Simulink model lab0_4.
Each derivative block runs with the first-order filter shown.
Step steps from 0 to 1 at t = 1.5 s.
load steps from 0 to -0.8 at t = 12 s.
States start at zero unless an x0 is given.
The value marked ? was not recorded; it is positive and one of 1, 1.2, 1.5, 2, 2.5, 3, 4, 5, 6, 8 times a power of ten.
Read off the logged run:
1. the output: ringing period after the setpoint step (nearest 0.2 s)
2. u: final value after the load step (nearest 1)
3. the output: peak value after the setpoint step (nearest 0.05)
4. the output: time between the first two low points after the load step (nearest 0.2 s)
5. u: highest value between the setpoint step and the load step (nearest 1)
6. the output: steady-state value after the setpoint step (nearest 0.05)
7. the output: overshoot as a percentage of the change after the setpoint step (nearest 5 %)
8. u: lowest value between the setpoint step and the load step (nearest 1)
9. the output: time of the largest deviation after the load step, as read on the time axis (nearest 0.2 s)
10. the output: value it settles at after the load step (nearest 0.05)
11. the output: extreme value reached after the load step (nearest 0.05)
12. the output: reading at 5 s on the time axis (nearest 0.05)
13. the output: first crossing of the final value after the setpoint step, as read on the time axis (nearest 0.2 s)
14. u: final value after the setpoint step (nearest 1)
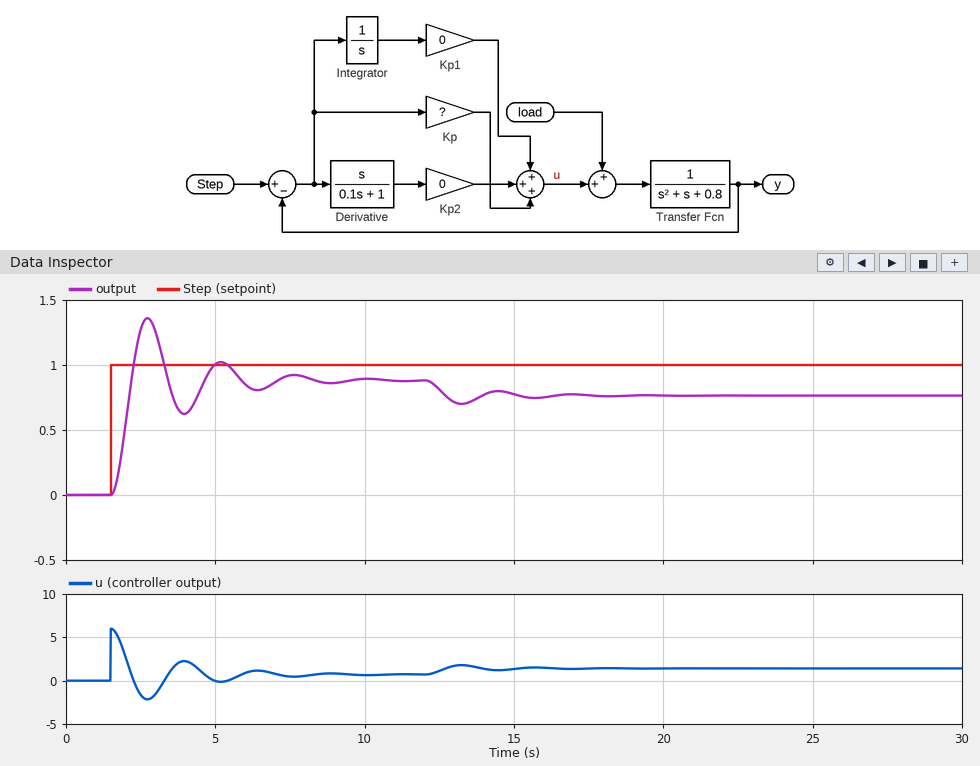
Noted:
2.4 s
1
1.35
2.4 s
6
0.90
55 %
-2
13.2 s
0.75
0.70
1.00
2.2 s
1
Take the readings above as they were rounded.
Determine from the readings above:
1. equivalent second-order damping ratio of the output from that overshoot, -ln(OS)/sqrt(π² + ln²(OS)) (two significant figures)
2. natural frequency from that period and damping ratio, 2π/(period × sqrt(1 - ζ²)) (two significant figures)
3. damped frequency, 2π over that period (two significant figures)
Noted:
0.19
2.7 rad/s
2.6 rad/s
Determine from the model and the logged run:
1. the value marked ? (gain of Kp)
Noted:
6
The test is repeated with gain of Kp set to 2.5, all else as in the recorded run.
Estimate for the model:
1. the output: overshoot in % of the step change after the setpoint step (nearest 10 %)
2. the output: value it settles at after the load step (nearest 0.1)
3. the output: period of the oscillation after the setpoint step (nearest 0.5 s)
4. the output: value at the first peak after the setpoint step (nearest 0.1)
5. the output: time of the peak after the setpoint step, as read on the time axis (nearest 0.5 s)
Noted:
40 %
0.5
3.5 s
1.1
3.5 s
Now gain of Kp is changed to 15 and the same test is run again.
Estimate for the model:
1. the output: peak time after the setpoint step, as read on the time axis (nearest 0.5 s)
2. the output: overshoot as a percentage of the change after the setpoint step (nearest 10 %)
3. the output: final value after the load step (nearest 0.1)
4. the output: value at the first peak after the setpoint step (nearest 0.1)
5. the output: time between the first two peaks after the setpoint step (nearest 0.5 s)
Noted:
2.5 s
70 %
0.9
1.6
1.5 s
